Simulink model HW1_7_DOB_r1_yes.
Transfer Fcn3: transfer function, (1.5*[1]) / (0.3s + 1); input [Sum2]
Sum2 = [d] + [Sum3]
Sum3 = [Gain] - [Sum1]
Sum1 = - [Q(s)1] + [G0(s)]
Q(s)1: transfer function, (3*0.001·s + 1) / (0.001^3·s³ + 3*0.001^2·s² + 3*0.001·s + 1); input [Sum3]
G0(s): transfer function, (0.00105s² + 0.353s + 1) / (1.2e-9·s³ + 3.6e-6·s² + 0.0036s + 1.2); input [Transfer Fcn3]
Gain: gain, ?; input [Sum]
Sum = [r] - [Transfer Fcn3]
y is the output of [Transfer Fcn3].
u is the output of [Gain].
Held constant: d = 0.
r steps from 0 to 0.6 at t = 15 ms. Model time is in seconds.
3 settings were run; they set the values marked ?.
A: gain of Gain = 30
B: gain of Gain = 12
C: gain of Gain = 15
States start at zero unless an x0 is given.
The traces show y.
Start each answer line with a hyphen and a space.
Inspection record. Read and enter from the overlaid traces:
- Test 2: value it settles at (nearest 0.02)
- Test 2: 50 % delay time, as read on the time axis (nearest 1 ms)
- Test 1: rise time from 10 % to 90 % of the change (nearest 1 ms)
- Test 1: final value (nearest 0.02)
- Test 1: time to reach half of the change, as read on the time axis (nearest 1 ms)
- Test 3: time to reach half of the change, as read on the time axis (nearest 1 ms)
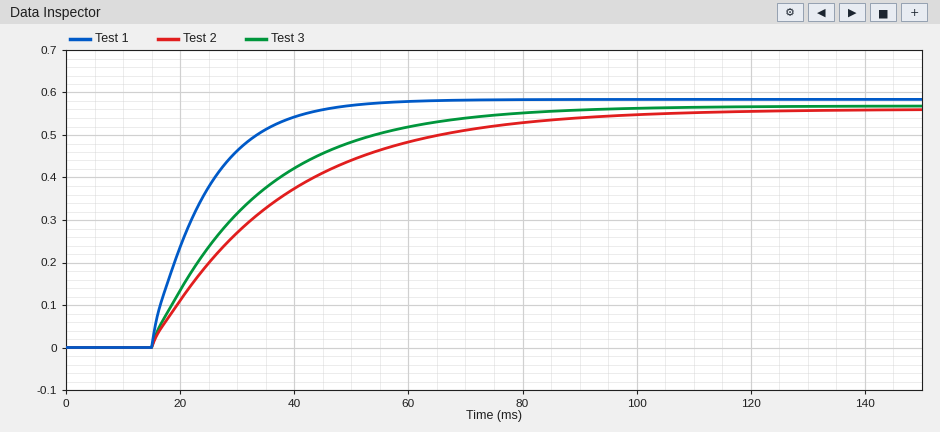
- 0.56
- 31 ms
- 21 ms
- 0.58
- 22 ms
- 28 ms
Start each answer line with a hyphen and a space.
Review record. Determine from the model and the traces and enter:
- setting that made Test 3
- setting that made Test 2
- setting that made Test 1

- C
- B
- A
